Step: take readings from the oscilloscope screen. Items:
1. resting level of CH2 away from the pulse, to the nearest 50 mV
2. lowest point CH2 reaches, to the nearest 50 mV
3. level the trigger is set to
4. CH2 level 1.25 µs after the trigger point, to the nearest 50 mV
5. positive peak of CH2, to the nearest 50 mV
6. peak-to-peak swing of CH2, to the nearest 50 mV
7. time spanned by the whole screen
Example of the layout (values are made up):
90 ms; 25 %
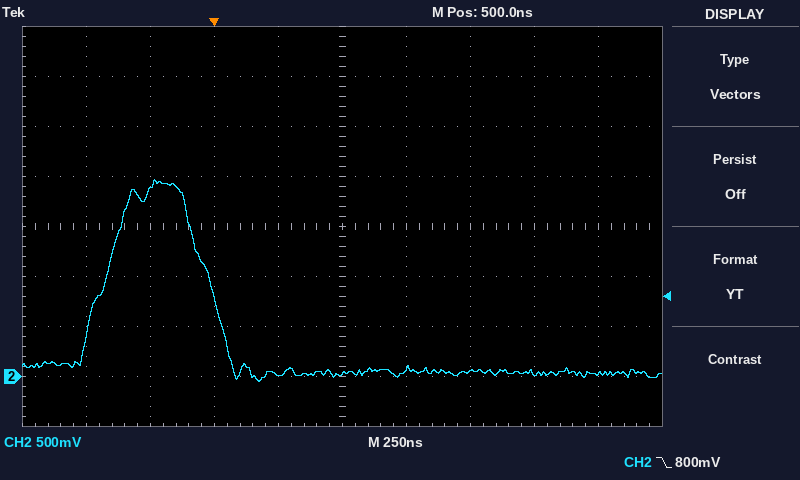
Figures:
50 mV; -50 mV; 800 mV; 50 mV; 1.95 V; 2.00 V; 2.5 µs
